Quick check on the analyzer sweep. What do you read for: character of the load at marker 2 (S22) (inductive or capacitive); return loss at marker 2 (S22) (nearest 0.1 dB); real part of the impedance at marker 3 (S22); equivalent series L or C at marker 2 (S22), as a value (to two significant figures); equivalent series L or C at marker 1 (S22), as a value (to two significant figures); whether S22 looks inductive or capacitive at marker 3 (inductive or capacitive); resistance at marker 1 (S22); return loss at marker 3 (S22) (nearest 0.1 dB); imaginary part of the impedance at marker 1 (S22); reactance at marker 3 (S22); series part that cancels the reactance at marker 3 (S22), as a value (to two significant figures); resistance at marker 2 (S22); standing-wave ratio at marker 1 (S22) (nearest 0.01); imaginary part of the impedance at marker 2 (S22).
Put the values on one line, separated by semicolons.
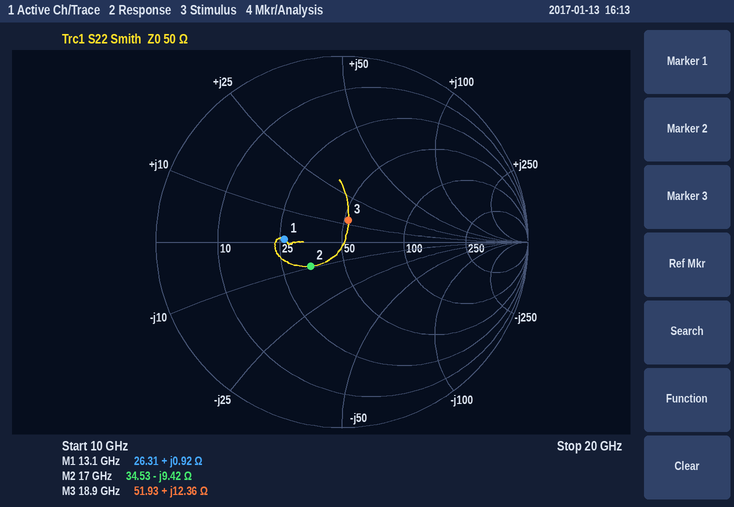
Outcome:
capacitive; 13.4 dB; 51.93 Ω; 990 fF; 11 pH; inductive; 26.31 Ω; 18.3 dB; +0.92 Ω; +12.36 Ω; 680 fF; 34.53 Ω; 1.90; -9.42 Ω
